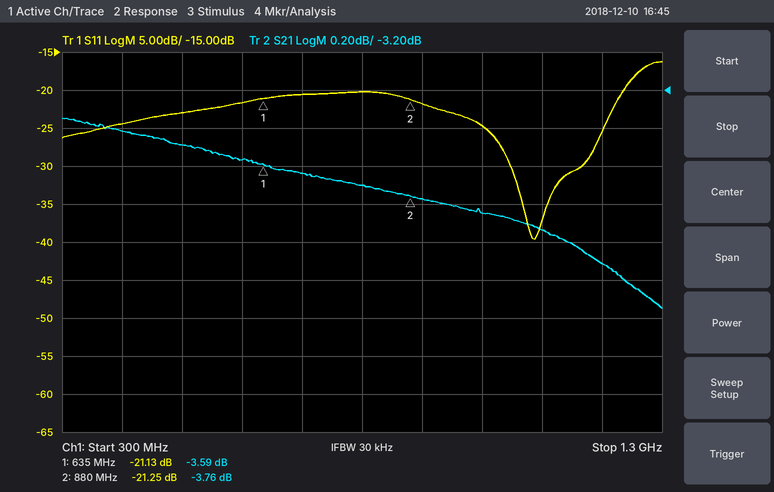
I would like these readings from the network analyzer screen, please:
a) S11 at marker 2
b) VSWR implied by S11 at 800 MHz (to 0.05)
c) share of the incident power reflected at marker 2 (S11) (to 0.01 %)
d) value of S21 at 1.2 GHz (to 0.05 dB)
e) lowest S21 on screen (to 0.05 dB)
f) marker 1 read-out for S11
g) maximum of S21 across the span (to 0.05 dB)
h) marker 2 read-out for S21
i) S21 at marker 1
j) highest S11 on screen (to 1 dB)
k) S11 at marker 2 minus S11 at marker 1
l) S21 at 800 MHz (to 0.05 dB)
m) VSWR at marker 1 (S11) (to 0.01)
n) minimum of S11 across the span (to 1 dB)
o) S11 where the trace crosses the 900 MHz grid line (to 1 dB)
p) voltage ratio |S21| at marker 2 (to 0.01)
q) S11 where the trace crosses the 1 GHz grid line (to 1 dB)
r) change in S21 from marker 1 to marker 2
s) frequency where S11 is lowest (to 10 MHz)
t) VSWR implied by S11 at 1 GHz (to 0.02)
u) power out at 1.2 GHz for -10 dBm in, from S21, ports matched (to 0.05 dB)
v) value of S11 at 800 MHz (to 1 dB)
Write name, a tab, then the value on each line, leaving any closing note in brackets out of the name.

S11 at marker 2	-21.25 dB
VSWR implied by S11 at 800 MHz	1.20
share of the incident power reflected at marker 2 (S11)	0.75 %
value of S21 at 1.2 GHz	-4.10 dB
lowest S21 on screen	-4.35 dB
marker 1 read-out for S11	-21.13 dB
maximum of S21 across the span	-3.35 dB
marker 2 read-out for S21	-3.76 dB
S21 at marker 1	-3.59 dB
highest S11 on screen	-16 dB
S11 at marker 2 minus S11 at marker 1	-0.12 dB
S21 at 800 MHz	-3.70 dB
VSWR at marker 1 (S11)	1.19
minimum of S11 across the span	-40 dB
S11 where the trace crosses the 900 MHz grid line	-22 dB
voltage ratio |S21| at marker 2	0.65
S11 where the trace crosses the 1 GHz grid line	-25 dB
change in S21 from marker 1 to marker 2	-0.17 dB
frequency where S11 is lowest	1.09 GHz
VSWR implied by S11 at 1 GHz	1.12
power out at 1.2 GHz for -10 dBm in, from S21, ports matched	-14.10 dBm
value of S11 at 800 MHz	-20 dB
